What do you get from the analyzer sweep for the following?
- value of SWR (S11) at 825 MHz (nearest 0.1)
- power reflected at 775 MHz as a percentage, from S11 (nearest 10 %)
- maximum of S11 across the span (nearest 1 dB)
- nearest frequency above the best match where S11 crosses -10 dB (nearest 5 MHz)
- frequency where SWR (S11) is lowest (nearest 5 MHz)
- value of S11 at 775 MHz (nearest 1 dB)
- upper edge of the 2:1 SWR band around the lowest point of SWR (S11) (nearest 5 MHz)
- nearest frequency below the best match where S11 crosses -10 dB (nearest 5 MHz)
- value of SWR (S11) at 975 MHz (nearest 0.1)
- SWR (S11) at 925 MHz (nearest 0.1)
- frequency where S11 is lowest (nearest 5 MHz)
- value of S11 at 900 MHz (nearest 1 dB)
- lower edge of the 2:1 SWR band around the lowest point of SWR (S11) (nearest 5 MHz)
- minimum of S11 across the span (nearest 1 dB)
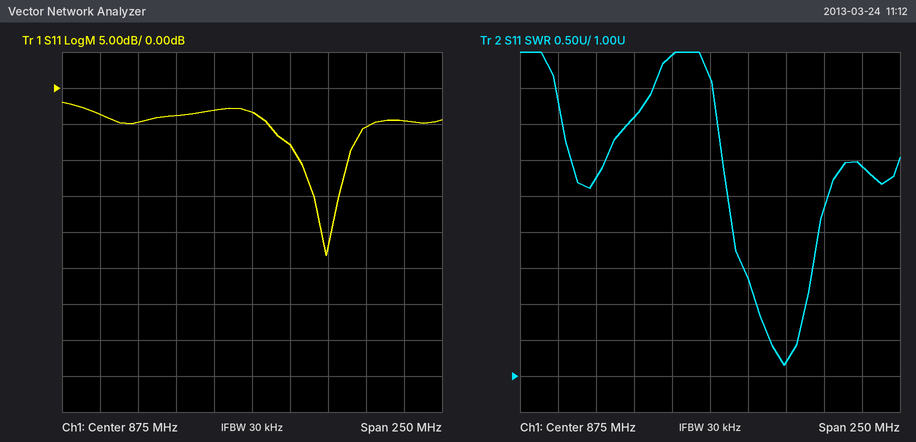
4.6
40 %
-2 dB
940 MHz
925 MHz
-4 dB
940 MHz
905 MHz
3.9
1.2
925 MHz
-8 dB
905 MHz
-23 dB
